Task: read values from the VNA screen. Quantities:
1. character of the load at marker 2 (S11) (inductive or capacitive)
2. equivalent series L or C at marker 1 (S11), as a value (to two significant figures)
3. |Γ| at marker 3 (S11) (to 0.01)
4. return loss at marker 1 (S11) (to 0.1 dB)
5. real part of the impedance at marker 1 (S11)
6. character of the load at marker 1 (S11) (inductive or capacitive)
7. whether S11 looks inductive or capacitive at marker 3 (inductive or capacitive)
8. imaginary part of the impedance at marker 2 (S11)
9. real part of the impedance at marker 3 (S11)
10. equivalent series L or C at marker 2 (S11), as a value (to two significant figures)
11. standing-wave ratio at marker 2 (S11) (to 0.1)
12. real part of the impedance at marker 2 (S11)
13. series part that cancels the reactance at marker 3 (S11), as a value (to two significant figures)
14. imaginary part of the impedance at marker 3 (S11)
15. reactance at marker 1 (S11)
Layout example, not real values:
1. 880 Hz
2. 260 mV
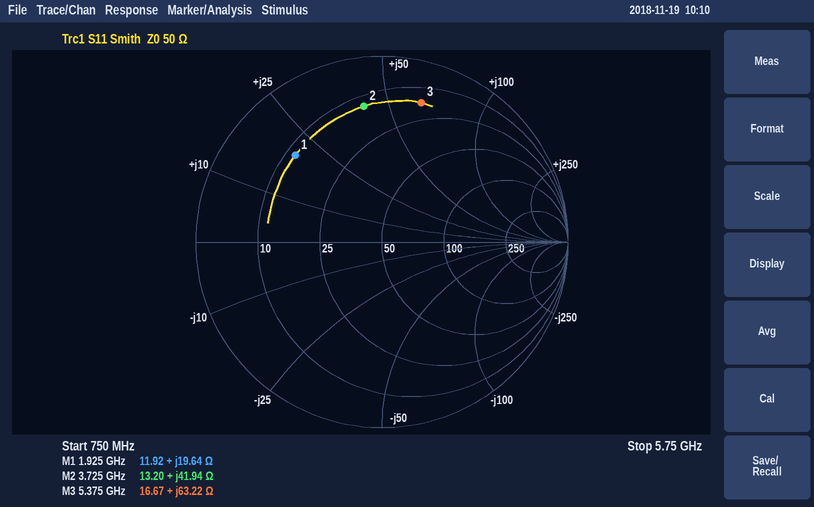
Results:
1. inductive
2. 1.6 nH
3. 0.78
4. 3.6 dB
5. 11.92 Ω
6. inductive
7. inductive
8. +41.94 Ω
9. 16.67 Ω
10. 1.8 nH
11. 6.6
12. 13.20 Ω
13. 470 fF
14. +63.22 Ω
15. +19.64 Ω
